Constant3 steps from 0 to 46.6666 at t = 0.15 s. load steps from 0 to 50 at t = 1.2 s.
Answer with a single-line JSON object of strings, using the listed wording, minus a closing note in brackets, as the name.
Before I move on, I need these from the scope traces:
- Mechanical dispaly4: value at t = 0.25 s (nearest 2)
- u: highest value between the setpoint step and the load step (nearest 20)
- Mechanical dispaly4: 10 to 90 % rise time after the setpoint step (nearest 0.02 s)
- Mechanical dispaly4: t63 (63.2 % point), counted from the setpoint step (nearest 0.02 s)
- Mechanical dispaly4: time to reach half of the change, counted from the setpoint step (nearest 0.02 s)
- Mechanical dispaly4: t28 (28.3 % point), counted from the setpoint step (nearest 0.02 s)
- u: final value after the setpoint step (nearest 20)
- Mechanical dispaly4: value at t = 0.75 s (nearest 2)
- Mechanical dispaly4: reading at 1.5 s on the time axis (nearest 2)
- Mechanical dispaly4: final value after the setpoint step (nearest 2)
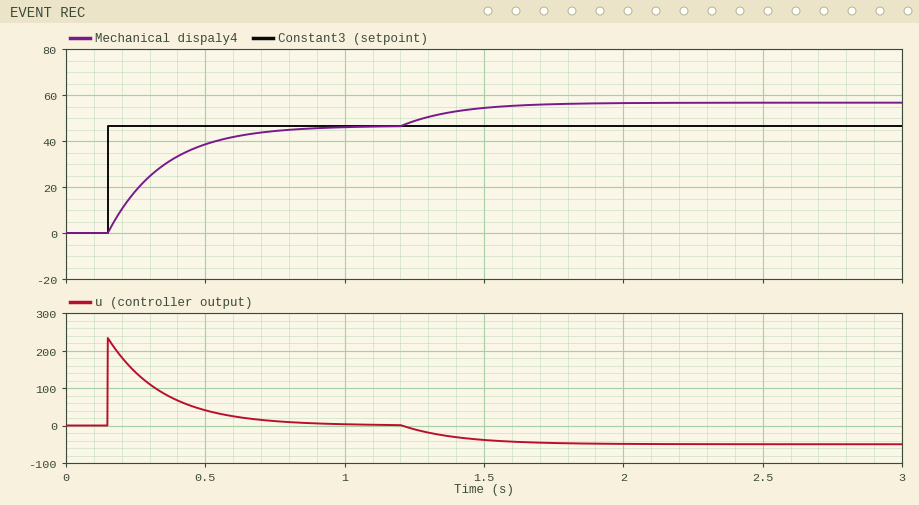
{"Mechanical dispaly4: value at t = 0.25 s": "18", "u: highest value between the setpoint step and the load step": "240", "Mechanical dispaly4: 10 to 90 % rise time after the setpoint step": "0.44 s", "Mechanical dispaly4: t63 (63.2 % point), counted from the setpoint step": "0.20 s", "Mechanical dispaly4: time to reach half of the change, counted from the setpoint step": "0.14 s", "Mechanical dispaly4: t28 (28.3 % point), counted from the setpoint step": "0.06 s", "u: final value after the setpoint step": "0", "Mechanical dispaly4: value at t = 0.75 s": "44", "Mechanical dispaly4: reading at 1.5 s on the time axis": "54", "Mechanical dispaly4: final value after the setpoint step": "46"}
